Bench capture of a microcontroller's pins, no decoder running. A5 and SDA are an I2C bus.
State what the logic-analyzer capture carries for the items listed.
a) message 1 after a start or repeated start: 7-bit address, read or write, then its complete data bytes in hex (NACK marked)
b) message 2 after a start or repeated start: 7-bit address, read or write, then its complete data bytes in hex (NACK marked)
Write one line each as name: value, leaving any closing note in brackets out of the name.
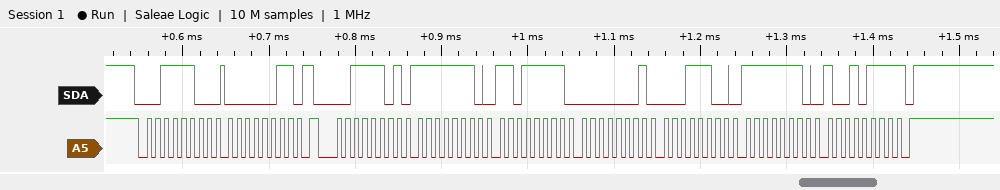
message 1 after a start or repeated start: 7-bit address, read or write, then its complete data bytes in hex: 0x1E write: 03
message 2 after a start or repeated start: 7-bit address, read or write, then its complete data bytes in hex: 0x1E read: FE DF 01 1C FE 97 NACK
